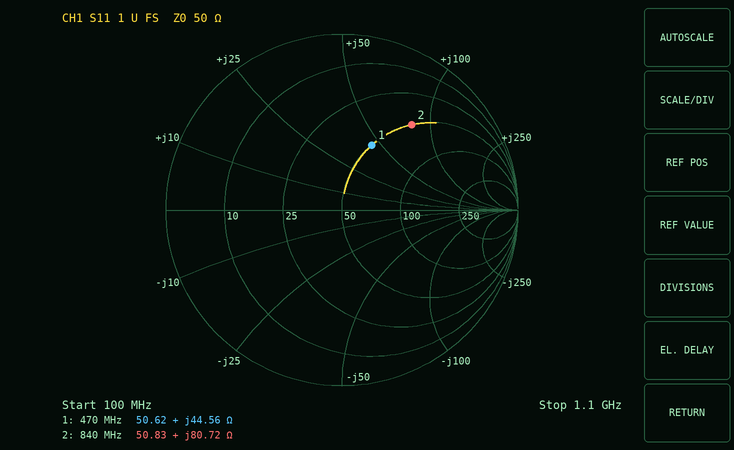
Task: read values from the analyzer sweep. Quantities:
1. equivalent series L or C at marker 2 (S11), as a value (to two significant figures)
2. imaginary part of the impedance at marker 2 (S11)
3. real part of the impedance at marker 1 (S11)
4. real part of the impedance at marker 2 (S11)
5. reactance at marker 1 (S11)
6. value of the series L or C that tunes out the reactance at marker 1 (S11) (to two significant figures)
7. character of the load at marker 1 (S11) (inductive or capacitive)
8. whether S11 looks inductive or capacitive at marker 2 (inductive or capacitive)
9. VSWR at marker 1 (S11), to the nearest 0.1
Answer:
15 nH
+80.72 Ω
50.62 Ω
50.83 Ω
+44.56 Ω
7.6 pF
inductive
inductive
2.4
